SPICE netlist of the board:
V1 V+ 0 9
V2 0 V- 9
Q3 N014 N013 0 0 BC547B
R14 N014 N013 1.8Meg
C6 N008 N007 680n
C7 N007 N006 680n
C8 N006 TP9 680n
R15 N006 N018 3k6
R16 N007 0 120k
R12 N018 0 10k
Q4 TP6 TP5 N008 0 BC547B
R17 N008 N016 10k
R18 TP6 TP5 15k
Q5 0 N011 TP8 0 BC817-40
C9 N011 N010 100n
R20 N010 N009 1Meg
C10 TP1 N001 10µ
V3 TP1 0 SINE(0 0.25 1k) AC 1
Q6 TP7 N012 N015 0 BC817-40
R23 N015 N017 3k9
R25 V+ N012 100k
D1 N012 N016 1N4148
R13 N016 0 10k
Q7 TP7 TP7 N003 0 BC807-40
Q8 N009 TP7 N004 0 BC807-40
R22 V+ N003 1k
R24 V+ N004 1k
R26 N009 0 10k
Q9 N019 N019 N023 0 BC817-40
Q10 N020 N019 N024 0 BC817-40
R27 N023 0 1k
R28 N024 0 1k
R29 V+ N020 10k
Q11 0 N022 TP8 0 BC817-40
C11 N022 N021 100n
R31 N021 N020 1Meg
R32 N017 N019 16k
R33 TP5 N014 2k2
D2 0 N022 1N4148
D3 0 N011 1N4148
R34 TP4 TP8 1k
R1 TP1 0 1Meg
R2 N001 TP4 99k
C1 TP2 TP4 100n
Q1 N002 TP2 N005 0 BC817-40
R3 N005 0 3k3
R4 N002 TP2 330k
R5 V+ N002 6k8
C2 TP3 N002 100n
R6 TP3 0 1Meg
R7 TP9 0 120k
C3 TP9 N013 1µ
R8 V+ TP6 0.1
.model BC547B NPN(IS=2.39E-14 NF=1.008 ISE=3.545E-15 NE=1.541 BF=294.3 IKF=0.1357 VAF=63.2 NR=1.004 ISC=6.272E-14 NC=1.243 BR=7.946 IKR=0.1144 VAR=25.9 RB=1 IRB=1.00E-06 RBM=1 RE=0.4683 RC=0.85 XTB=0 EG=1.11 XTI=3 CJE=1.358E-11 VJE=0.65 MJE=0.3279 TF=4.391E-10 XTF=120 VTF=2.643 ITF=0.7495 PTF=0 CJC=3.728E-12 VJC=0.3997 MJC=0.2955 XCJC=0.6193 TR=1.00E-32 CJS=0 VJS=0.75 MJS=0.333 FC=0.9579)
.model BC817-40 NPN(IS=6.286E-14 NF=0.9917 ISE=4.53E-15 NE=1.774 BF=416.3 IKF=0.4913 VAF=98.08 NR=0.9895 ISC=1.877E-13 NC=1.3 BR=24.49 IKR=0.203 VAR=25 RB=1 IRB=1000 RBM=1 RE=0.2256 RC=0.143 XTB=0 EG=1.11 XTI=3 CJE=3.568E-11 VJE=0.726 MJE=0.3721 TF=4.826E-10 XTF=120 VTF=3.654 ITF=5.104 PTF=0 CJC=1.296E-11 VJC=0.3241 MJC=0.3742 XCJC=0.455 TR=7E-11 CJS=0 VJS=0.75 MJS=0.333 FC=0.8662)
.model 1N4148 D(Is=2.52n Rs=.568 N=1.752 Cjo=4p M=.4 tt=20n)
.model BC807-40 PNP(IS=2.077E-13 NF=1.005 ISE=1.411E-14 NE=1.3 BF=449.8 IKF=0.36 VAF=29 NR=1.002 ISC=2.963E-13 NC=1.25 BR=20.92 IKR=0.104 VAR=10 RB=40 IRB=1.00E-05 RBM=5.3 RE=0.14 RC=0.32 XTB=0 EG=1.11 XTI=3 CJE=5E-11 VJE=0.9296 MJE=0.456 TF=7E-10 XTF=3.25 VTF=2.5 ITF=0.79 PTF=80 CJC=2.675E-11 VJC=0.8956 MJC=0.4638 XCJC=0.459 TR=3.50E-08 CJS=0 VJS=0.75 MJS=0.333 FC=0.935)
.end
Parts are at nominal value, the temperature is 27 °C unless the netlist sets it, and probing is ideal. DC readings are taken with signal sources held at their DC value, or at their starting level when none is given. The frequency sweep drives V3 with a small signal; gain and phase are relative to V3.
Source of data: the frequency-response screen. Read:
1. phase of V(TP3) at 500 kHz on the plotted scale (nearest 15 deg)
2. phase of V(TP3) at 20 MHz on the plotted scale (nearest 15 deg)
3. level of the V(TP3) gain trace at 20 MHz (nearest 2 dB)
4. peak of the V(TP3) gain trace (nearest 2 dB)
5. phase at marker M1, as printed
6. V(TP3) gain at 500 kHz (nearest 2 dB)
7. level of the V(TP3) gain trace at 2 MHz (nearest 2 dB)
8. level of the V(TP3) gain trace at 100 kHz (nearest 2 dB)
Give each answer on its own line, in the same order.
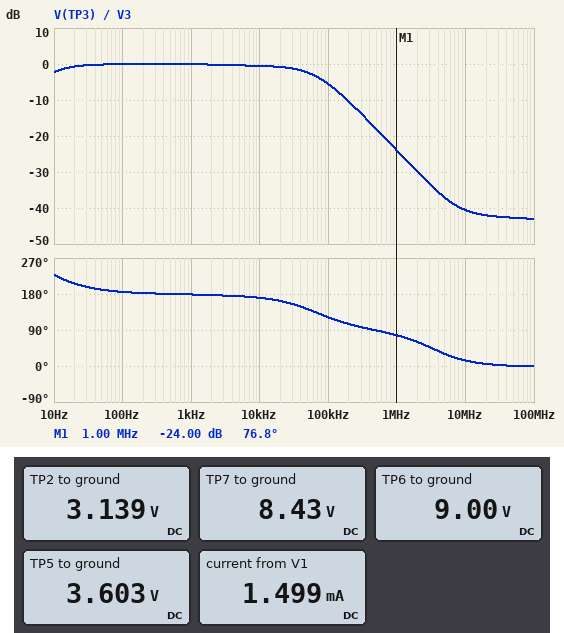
90 deg
0 deg
-42 dB
0 dB
76.8 deg
-18 dB
-30 dB
-6 dB
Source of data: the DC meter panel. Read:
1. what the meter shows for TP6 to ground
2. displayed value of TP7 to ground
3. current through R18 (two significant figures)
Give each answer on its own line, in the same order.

9.00 V
8.43 V
360 µA
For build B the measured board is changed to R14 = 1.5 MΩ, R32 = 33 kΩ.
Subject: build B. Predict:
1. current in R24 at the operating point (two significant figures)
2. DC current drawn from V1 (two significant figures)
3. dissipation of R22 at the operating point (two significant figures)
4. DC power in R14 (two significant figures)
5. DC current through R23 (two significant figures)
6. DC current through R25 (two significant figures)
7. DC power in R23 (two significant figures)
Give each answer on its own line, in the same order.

34 µA
1.4 mA
940 nW
2.5 µW
31 µA
68 µA
3.7 µW
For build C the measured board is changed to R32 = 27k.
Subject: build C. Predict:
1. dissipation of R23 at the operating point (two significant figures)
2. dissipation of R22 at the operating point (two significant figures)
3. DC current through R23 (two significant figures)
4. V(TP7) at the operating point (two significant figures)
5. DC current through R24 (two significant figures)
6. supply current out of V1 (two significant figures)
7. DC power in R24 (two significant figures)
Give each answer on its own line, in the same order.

6.2 µW
1.6 µW
40 µA
8.5 V
44 µA
1.4 mA
1.9 µW
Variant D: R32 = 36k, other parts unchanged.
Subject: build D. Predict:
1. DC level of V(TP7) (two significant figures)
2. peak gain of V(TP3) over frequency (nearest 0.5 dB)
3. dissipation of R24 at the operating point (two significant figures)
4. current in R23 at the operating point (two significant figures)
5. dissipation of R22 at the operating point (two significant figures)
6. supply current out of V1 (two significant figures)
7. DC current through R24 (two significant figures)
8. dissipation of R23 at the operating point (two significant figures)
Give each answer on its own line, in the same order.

8.5 V
0 dB
1.2 µW
31 µA
970 nW
1.4 mA
35 µA
3.8 µW
